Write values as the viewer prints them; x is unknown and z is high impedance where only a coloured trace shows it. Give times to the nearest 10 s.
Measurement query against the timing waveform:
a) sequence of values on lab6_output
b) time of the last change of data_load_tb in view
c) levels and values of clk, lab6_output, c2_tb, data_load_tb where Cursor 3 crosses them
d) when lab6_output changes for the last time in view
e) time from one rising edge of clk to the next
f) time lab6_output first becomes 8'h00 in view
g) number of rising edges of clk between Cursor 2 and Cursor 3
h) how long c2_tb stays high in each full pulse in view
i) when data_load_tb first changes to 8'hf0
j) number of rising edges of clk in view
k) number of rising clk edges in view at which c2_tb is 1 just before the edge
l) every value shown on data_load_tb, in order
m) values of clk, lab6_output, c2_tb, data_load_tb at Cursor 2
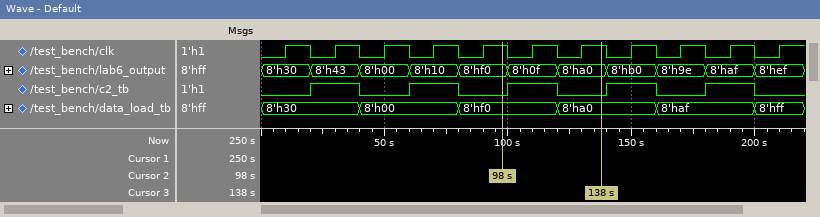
8'h30, 8'h43, 8'h00, 8'h10, 8'hf0, 8'h0f, 8'ha0, 8'hb0, 8'h9e, 8'haf, 8'hef
200 s
clk=1, lab6_output=8'ha0, c2_tb=0, data_load_tb=8'ha0
200 s
20 s
40 s
2
20 s, 20 s, 20 s, 20 s, 20 s
80 s
11
5
8'h30, 8'h00, 8'hf0, 8'ha0, 8'haf, 8'hff
clk=1, lab6_output=8'hf0, c2_tb=0, data_load_tb=8'hf0
